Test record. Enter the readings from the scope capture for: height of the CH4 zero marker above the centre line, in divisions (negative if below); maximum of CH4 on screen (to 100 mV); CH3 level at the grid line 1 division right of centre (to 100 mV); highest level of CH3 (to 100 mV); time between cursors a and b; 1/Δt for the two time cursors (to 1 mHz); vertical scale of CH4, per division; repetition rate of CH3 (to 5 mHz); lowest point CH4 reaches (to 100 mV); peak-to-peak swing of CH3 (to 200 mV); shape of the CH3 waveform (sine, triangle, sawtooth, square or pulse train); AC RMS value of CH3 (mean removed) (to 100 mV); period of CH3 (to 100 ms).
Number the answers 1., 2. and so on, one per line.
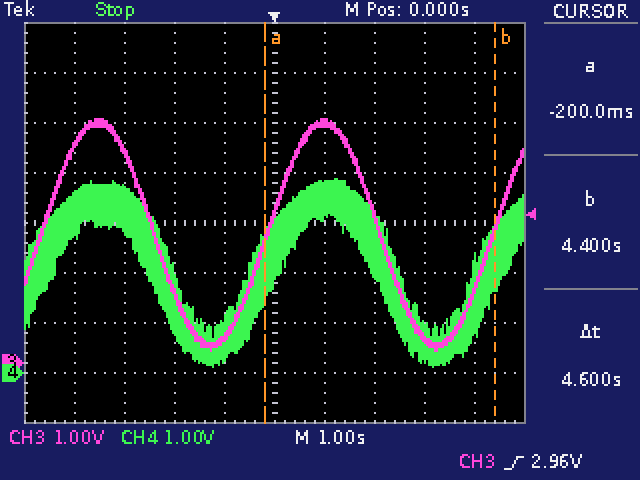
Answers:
1. -3.0 div
2. 3.9 V
3. 4.8 V
4. 4.9 V
5. 4.6 s
6. 217 mHz
7. 1 V
8. 220 mHz
9. 100 mV
10. 4.6 V
11. sine
12. 1.6 V
13. 4.5 s
